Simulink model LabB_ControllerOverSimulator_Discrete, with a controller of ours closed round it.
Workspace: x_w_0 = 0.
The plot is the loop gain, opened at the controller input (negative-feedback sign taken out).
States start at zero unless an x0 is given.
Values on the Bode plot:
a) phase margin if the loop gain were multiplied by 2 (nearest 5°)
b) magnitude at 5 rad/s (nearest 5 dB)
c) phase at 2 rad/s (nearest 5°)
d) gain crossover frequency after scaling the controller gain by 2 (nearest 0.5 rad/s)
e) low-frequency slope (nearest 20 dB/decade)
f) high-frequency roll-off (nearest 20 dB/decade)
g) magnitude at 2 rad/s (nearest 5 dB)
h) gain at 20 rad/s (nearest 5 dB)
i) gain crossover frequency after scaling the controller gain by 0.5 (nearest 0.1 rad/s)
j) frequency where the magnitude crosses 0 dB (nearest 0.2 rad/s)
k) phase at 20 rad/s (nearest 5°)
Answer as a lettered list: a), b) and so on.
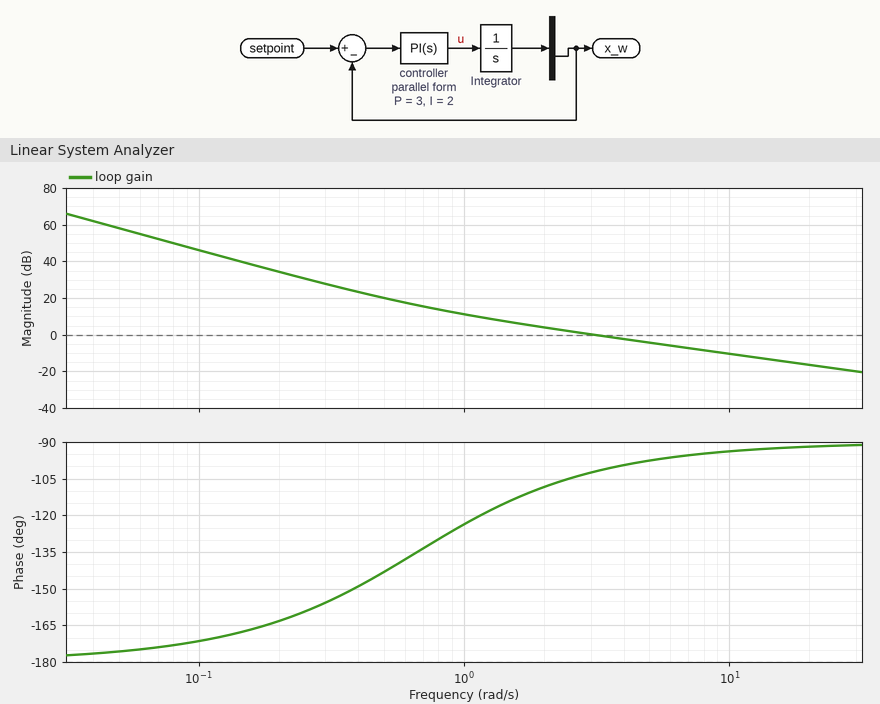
a) 85°
b) -5 dB
c) -110°
d) 6.0 rad/s
e) -40 dB/decade
f) -20 dB/decade
g) 5 dB
h) -15 dB
i) 1.6 rad/s
j) 3.0 rad/s
k) -90°
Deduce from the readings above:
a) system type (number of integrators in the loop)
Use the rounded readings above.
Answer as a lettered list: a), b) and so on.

a) 2
